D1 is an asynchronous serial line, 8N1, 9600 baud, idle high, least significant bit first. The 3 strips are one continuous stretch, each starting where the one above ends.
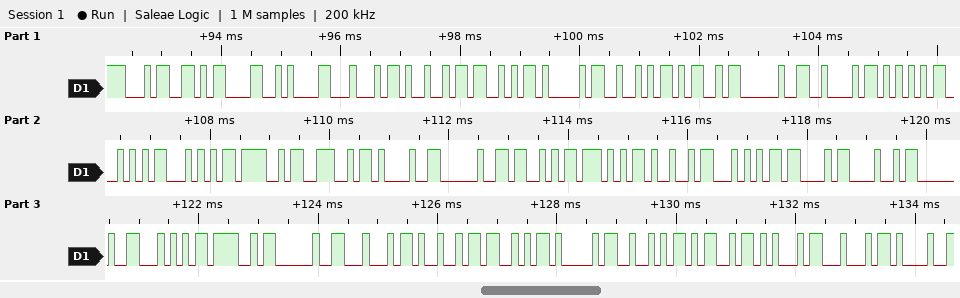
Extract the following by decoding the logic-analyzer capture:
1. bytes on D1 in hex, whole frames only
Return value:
34 0D 0A 44 49 53 41 52 4D 20 42 55 54 54 4F 4E 21 20 53 57 49 54 43 48 20 54 4F 20 44 49 53 41 52 4D 45 44 21
